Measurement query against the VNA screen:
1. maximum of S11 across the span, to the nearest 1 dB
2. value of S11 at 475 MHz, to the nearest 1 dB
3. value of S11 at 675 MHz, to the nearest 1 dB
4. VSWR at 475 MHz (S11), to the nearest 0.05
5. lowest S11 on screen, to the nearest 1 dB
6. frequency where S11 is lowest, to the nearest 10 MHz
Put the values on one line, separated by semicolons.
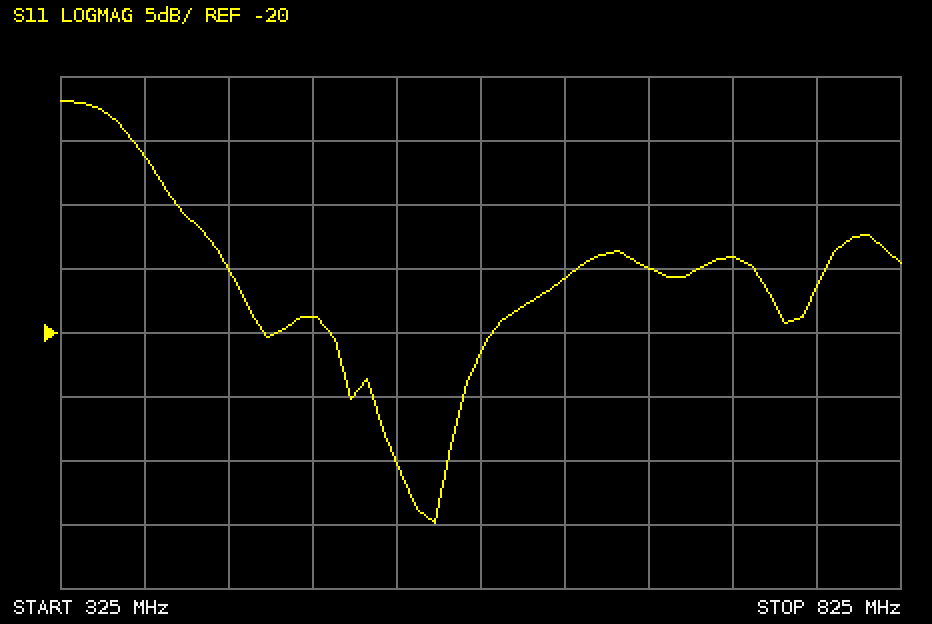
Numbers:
-2 dB; -19 dB; -15 dB; 1.25; -35 dB; 550 MHz
